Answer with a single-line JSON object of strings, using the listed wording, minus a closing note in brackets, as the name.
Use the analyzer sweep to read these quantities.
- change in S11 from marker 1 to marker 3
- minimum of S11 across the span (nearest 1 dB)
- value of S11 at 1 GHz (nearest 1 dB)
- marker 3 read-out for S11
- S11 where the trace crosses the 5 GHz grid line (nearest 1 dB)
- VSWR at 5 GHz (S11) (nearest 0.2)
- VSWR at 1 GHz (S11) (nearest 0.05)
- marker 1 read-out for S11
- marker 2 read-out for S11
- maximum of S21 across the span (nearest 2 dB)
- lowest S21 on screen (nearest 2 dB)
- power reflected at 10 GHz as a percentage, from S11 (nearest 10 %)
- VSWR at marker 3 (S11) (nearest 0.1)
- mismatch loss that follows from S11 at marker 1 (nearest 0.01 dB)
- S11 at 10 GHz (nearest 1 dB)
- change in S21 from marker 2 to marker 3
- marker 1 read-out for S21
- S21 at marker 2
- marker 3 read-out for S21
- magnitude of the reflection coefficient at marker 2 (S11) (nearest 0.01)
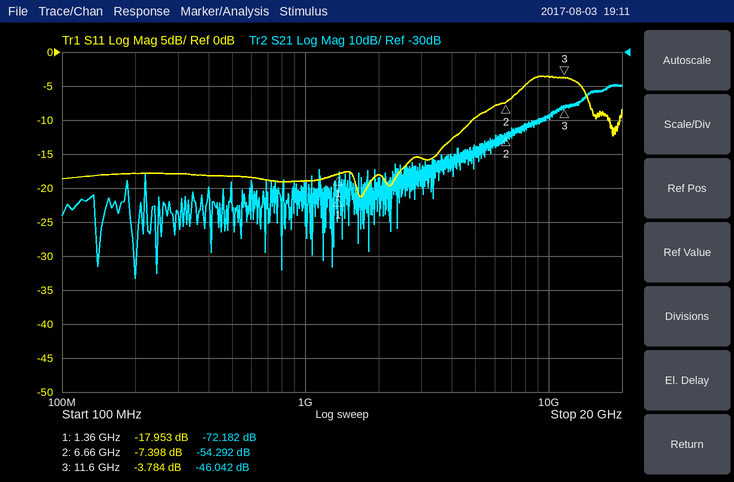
{"change in S11 from marker 1 to marker 3": "14.169 dB", "minimum of S11 across the span": "-21 dB", "value of S11 at 1 GHz": "-19 dB", "marker 3 read-out for S11": "-3.784 dB", "S11 where the trace crosses the 5 GHz grid line": "-10 dB", "VSWR at 5 GHz (S11)": "2.0", "VSWR at 1 GHz (S11)": "1.25", "marker 1 read-out for S11": "-17.953 dB", "marker 2 read-out for S11": "-7.398 dB", "maximum of S21 across the span": "-40 dB", "lowest S21 on screen": "-96 dB", "power reflected at 10 GHz as a percentage, from S11": "40 %", "VSWR at marker 3 (S11)": "4.7", "mismatch loss that follows from S11 at marker 1": "0.07 dB", "S11 at 10 GHz": "-4 dB", "change in S21 from marker 2 to marker 3": "8.250 dB", "marker 1 read-out for S21": "-72.182 dB", "S21 at marker 2": "-54.292 dB", "marker 3 read-out for S21": "-46.042 dB", "magnitude of the reflection coefficient at marker 2 (S11)": "0.43"}
